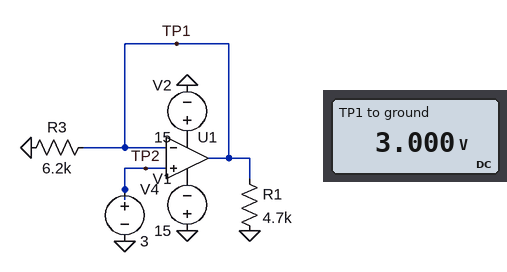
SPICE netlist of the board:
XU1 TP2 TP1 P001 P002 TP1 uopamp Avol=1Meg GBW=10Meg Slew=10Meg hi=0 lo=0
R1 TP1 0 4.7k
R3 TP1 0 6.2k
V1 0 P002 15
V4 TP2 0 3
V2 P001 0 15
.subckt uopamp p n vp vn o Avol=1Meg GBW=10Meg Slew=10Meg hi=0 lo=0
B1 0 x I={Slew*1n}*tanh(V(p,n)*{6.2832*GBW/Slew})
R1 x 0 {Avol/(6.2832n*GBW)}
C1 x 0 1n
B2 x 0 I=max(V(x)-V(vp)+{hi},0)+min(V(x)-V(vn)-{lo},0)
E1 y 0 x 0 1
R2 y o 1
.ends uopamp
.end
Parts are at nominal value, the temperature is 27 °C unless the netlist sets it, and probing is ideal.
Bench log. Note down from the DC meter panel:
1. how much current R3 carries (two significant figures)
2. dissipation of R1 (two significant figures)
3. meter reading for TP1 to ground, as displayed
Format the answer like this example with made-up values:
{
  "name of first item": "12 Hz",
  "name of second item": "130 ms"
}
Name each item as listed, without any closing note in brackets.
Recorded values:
{
  "how much current R3 carries": "480 µA",
  "dissipation of R1": "1.9 mW",
  "meter reading for TP1 to ground, as displayed": "3.000 V"
}
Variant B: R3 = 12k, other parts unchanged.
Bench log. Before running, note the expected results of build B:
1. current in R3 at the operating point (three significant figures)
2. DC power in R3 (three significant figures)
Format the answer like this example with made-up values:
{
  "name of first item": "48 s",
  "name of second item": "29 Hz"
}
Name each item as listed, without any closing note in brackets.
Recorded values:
{
  "current in R3 at the operating point": "250 µA",
  "DC power in R3": "750 µW"
}
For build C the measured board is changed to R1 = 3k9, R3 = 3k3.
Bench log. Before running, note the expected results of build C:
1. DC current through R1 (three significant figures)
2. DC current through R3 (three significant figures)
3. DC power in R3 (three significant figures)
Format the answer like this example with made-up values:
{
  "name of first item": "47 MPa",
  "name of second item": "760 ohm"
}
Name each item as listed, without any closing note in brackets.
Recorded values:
{
  "DC current through R1": "769 µA",
  "DC current through R3": "909 µA",
  "DC power in R3": "2.73 mW"
}
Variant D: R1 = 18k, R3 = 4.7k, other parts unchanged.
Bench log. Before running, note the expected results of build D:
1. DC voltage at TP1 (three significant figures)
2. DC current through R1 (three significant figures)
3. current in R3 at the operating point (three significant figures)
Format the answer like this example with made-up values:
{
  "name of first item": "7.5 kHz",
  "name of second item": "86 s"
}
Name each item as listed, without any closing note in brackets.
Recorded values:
{
  "DC voltage at TP1": "3.00 V",
  "DC current through R1": "167 µA",
  "current in R3 at the operating point": "638 µA"
}
